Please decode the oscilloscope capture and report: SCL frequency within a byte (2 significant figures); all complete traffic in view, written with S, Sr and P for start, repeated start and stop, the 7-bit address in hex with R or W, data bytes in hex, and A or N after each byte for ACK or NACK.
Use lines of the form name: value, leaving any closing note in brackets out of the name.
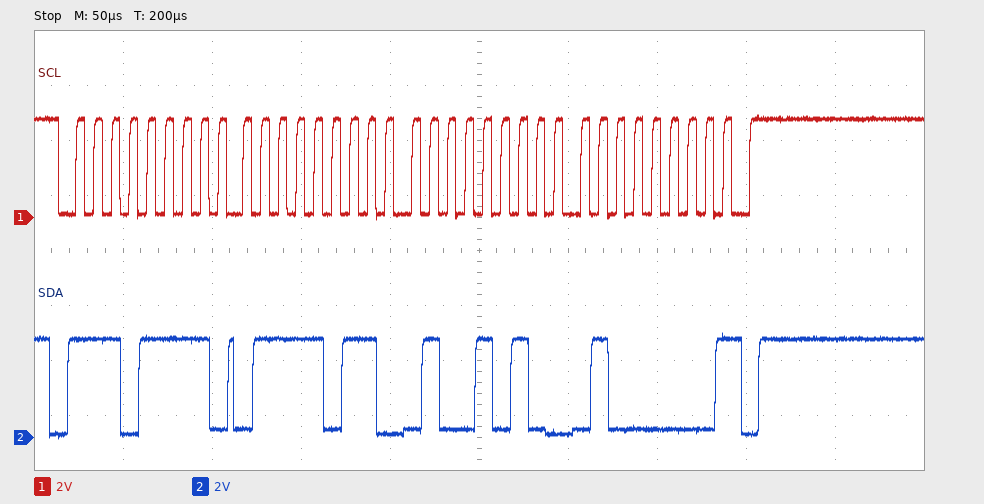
SCL frequency within a byte: 100 kHz
all complete traffic in view, written with S, Sr and P for start, repeated start and stop, the 7-bit address in hex with R or W, data bytes in hex, and A or N after each byte for ACK or NACK: S 77R A 7B A 4A A 40 N P
